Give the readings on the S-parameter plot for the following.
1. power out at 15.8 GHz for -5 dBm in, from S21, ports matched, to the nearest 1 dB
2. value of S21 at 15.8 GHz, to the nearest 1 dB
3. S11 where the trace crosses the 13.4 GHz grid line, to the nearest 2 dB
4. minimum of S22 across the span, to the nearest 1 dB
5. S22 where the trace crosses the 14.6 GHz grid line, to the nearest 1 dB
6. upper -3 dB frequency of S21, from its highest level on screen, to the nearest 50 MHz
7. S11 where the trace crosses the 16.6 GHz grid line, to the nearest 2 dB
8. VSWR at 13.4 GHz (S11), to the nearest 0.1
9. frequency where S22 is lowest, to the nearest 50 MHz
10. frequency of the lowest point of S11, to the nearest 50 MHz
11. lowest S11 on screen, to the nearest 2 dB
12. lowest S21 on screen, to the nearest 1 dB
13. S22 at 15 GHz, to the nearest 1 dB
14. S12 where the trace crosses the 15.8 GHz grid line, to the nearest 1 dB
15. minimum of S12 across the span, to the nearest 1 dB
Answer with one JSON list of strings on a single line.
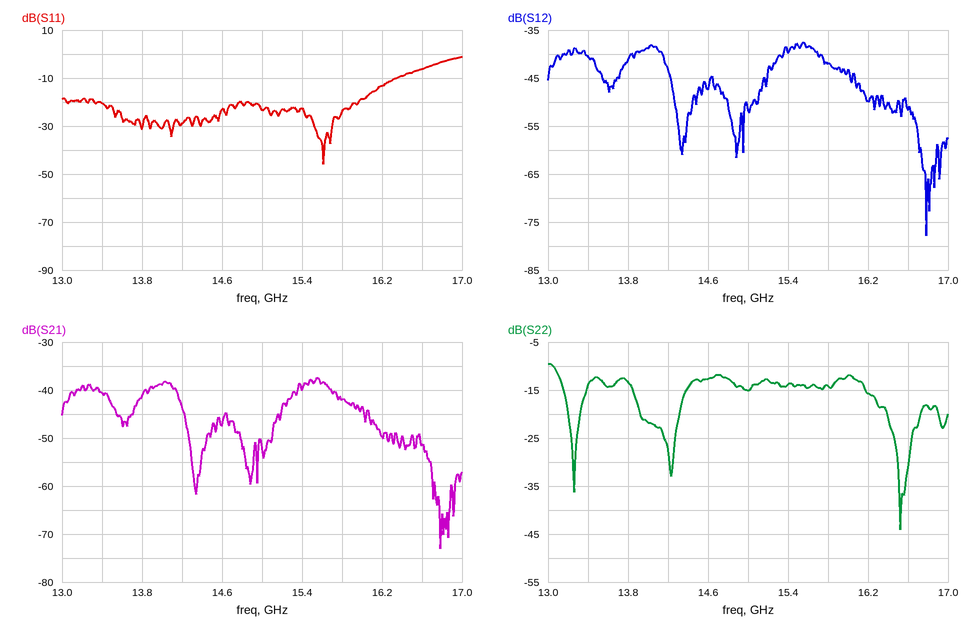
["-47 dBm", "-42 dB", "-20 dB", "-44 dB", "-13 dB", "15.70 GHz", "-6 dB", "1.2", "16.50 GHz", "15.60 GHz", "-46 dB", "-73 dB", "-15 dB", "-42 dB", "-78 dB"]
